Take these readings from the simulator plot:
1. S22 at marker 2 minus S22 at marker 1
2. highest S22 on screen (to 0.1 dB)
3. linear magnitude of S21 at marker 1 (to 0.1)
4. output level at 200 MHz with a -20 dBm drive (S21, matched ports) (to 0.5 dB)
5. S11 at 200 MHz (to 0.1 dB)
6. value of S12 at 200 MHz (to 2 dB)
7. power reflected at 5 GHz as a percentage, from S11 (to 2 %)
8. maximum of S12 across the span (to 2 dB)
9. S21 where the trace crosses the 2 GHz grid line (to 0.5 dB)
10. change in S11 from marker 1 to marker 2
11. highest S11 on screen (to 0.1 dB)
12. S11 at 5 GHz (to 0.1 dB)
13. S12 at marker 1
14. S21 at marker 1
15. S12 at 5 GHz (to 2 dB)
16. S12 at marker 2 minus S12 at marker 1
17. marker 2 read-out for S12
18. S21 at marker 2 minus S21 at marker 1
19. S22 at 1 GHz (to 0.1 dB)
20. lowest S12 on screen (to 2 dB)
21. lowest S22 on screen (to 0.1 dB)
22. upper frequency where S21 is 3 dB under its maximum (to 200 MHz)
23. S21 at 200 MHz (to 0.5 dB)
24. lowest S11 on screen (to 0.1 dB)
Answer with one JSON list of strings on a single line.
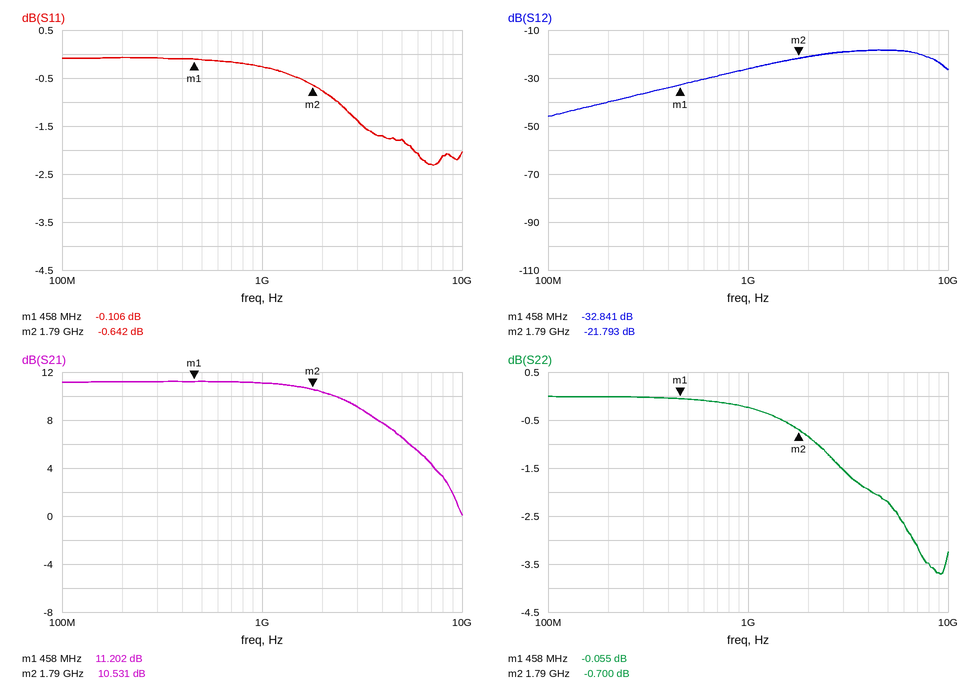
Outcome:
["-0.645 dB", "0.0 dB", "3.6", "-9.0 dBm", "-0.1 dB", "-40 dB", "66 %", "-18 dB", "10.5 dB", "-0.536 dB", "-0.1 dB", "-1.8 dB", "-32.841 dB", "11.202 dB", "-18 dB", "11.048 dB", "-21.793 dB", "-0.671 dB", "-0.2 dB", "-46 dB", "-3.7 dB", "3.6 GHz", "11.0 dB", "-2.3 dB"]
